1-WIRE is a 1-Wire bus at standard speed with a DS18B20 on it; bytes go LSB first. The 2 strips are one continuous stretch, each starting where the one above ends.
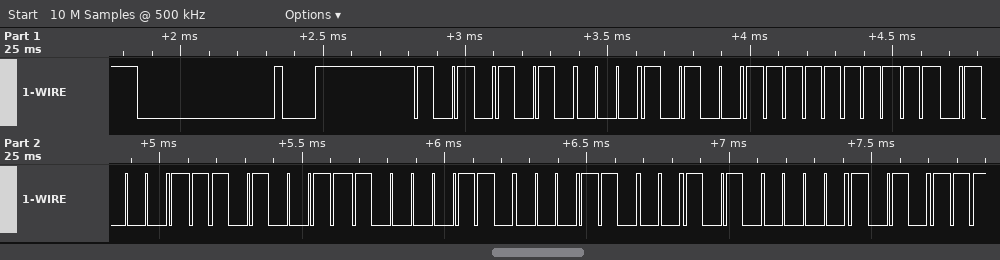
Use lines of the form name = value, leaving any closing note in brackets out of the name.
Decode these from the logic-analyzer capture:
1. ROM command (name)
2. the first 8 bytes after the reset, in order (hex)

ROM command = Match ROM
the first 8 bytes after the reset, in order = 55 28 FF 8B CB 61 18 05
